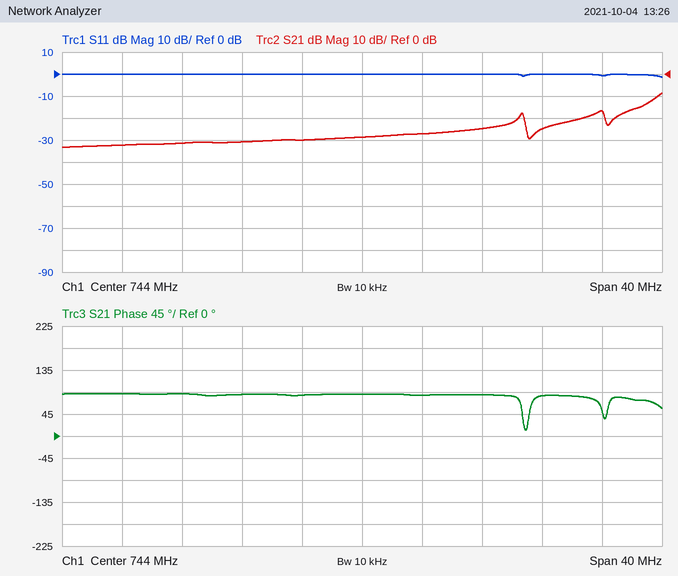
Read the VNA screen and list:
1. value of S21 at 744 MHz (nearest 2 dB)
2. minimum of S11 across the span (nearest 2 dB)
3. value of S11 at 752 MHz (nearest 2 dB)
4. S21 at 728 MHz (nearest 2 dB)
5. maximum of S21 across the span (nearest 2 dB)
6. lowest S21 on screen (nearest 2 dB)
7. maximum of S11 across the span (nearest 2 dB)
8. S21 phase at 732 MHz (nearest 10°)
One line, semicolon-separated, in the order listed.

-28 dB; -2 dB; 0 dB; -32 dB; -8 dB; -34 dB; 0 dB; 90°
